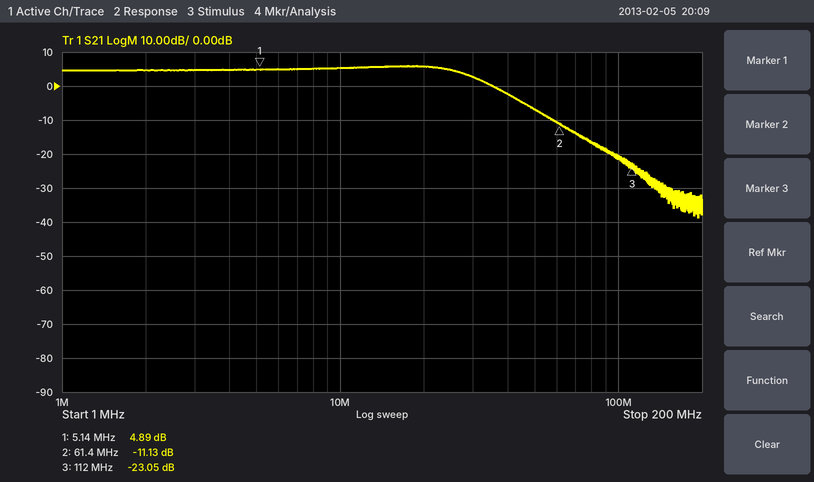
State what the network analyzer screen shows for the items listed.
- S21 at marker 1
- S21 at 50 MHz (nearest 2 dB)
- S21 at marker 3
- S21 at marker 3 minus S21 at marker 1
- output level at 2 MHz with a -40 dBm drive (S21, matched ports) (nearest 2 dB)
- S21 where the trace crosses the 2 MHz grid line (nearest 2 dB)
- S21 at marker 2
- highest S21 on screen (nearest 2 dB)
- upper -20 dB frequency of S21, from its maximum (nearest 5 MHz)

4.89 dB
-6 dB
-23.05 dB
-27.94 dB
-36 dBm
4 dB
-11.13 dB
6 dB
70 MHz
